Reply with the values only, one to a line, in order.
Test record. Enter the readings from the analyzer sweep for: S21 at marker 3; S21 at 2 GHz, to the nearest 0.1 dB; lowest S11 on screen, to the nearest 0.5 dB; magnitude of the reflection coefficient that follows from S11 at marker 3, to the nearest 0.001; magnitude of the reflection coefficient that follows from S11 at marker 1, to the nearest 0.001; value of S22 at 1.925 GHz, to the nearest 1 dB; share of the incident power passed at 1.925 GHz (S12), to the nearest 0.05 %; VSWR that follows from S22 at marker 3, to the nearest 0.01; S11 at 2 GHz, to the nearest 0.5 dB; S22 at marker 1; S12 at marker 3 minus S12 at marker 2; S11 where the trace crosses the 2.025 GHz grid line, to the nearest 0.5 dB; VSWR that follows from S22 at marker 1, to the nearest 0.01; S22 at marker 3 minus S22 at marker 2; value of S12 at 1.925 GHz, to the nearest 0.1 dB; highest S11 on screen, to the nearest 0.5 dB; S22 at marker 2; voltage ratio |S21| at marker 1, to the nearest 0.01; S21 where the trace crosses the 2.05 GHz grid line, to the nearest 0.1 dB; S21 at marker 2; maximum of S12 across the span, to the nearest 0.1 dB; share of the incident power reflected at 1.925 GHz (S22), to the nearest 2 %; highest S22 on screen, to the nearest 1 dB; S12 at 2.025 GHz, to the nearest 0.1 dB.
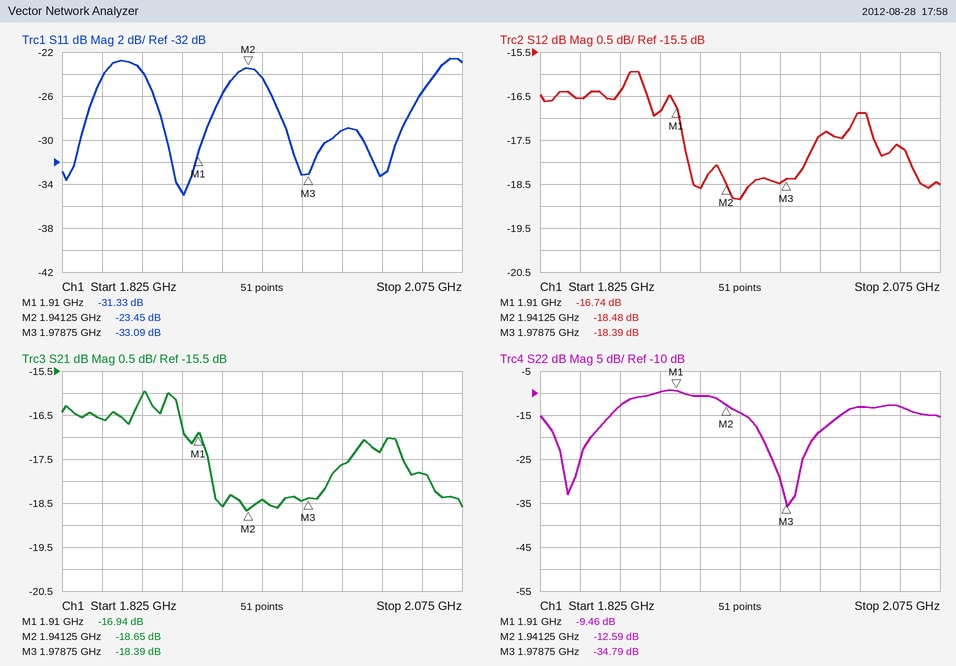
-18.39 dB
-17.6 dB
-35.0 dB
0.022
0.027
-11 dB
1.40 %
1.04
-29.0 dB
-9.46 dB
0.09 dB
-33.0 dB
2.01
-22.20 dB
-18.6 dB
-22.5 dB
-12.59 dB
0.14
-17.8 dB
-18.65 dB
-15.9 dB
8 %
-9 dB
-16.9 dB
